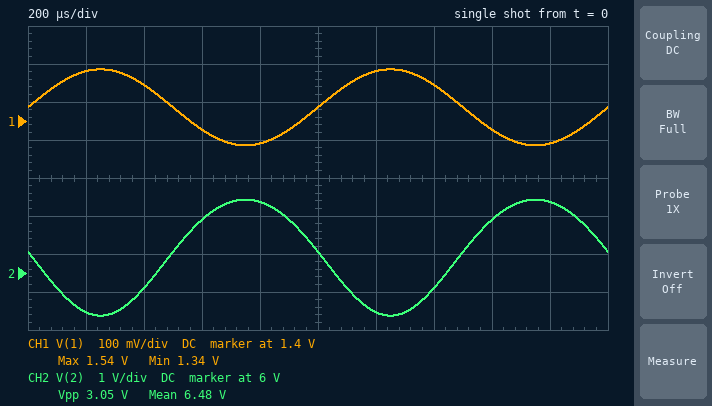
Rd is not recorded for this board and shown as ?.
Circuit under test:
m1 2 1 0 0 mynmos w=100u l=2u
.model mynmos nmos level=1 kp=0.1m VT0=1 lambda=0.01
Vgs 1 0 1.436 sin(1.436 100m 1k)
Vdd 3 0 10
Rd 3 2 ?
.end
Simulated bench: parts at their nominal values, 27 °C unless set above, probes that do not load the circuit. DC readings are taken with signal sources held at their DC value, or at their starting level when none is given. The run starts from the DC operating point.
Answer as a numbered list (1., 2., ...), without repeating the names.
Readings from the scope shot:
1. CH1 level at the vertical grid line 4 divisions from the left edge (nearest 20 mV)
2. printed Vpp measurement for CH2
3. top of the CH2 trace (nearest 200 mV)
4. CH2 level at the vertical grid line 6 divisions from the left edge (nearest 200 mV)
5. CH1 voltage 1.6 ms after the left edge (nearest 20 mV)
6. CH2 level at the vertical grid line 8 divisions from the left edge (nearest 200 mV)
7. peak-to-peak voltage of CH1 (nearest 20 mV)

1. 1.34 V
2. 3.05 V
3. 8.0 V
4. 5.0 V
5. 1.38 V
6. 7.4 V
7. 200 mV
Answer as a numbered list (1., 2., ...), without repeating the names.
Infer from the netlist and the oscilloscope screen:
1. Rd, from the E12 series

1. 6.8 kΩ
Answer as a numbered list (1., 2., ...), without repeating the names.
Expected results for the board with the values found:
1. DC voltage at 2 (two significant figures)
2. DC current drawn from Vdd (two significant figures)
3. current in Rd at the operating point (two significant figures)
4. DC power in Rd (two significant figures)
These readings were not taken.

1. 6.6 V
2. 510 µA
3. 510 µA
4. 1.7 mW
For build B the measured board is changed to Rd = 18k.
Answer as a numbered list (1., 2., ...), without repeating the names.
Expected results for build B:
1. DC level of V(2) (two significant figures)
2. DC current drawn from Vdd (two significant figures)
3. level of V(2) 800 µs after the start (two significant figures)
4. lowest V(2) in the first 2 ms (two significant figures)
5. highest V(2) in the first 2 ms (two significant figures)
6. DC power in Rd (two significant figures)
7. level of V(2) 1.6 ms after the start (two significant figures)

1. 1.3 V
2. 480 µA
3. 4.5 V
4. 270 mV
5. 4.7 V
6. 4.2 mW
7. 3.4 V
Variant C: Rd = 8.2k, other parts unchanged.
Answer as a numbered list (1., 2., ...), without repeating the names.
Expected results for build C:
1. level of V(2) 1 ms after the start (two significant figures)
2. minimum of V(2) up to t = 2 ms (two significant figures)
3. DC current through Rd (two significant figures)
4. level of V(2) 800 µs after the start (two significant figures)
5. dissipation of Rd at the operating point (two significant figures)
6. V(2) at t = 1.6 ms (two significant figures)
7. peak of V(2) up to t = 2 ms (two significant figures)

1. 5.9 V
2. 3.9 V
3. 500 µA
4. 7.4 V
5. 2.1 mW
6. 6.9 V
7. 7.5 V
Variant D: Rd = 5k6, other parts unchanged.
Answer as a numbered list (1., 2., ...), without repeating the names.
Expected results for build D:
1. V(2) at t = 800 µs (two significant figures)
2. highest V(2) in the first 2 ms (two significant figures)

1. 8.2 V
2. 8.3 V
